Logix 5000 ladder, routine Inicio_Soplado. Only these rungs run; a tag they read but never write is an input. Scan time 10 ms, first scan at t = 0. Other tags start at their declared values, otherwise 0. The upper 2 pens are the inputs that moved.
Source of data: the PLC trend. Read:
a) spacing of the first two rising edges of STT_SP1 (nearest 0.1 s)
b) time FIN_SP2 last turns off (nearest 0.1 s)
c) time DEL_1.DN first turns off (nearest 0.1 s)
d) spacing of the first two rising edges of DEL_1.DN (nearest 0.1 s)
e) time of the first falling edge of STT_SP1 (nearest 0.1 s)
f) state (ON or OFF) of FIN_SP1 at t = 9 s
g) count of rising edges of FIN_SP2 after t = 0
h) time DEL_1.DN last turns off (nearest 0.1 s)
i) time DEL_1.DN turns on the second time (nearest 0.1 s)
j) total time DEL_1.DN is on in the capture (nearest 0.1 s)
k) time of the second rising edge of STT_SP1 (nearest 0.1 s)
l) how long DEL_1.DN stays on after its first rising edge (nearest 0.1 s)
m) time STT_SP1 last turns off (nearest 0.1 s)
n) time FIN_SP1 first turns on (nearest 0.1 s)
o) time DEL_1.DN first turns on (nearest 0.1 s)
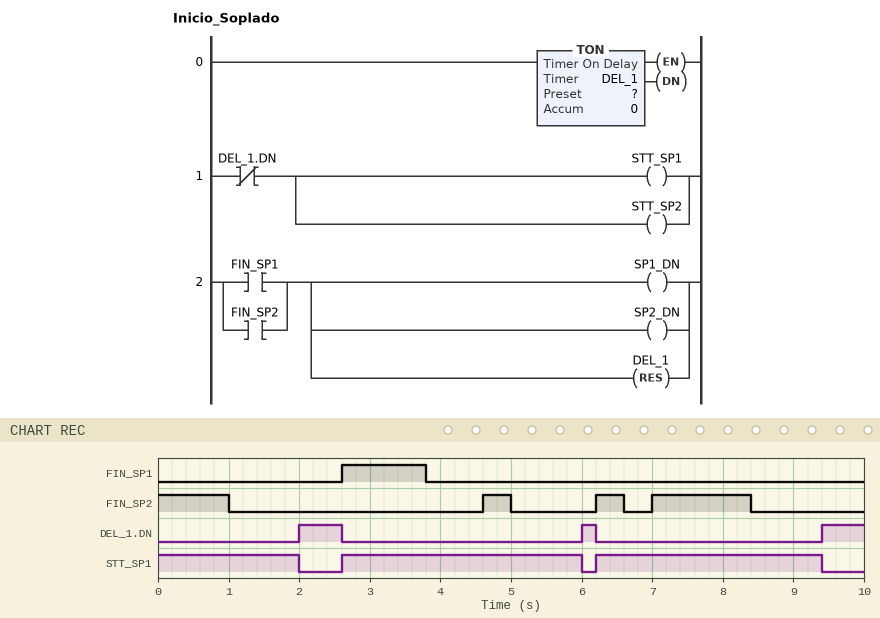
3.6 s
8.4 s
2.6 s
4.0 s
2.0 s
OFF
3
6.2 s
6.0 s
1.4 s
6.2 s
0.6 s
9.4 s
2.6 s
2.0 s
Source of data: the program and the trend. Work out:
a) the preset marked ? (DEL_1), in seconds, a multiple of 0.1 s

1.0 s
